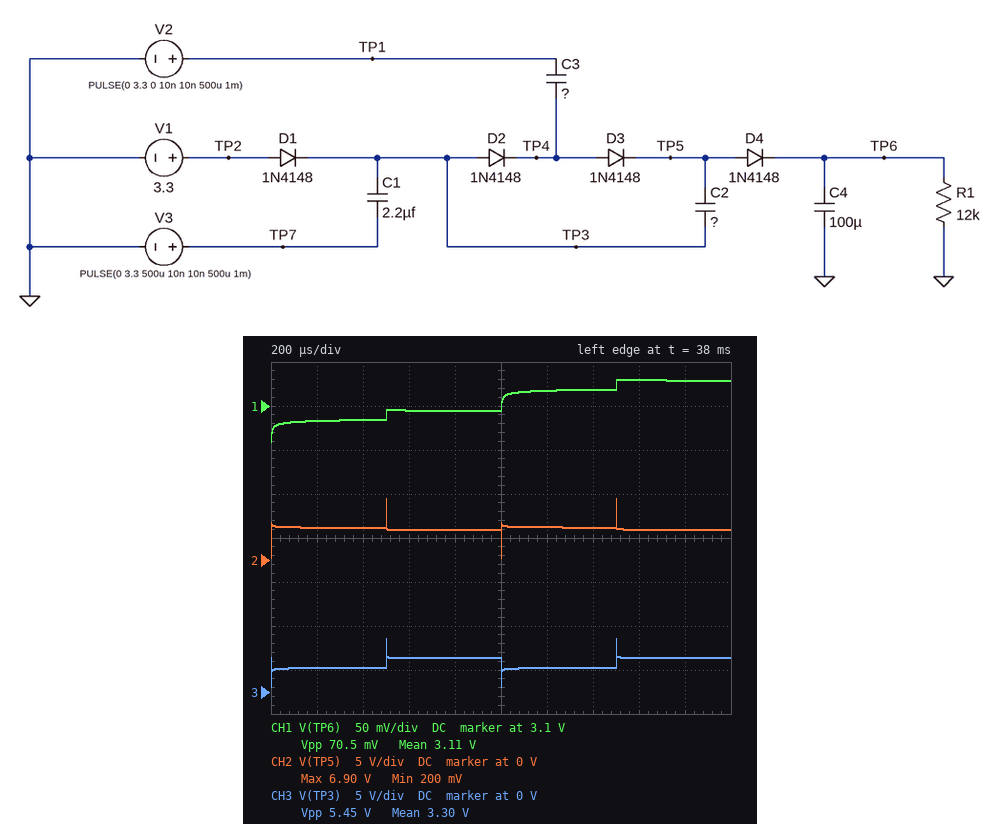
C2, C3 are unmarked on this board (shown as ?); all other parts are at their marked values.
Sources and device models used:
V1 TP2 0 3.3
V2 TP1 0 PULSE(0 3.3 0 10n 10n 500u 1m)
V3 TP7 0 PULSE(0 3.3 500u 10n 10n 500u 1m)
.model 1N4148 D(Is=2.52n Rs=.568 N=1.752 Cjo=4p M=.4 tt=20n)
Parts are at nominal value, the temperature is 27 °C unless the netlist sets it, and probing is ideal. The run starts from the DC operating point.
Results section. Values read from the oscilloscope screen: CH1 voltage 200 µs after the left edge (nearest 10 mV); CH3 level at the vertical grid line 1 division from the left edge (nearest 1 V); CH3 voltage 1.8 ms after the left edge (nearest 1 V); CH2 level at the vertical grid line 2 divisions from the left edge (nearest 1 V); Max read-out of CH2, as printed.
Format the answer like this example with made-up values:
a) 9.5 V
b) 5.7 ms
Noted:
a) 3.08 V
b) 3 V
c) 4 V
d) 4 V
e) 6.90 V
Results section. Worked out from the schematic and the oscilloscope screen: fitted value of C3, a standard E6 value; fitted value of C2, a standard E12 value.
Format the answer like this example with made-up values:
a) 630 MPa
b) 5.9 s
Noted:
a) 1.5 µF
b) 820 nF
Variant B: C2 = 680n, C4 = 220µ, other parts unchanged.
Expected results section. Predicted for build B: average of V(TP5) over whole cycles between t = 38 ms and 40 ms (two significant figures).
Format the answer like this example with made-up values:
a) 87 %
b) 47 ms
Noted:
a) 2.7 V
